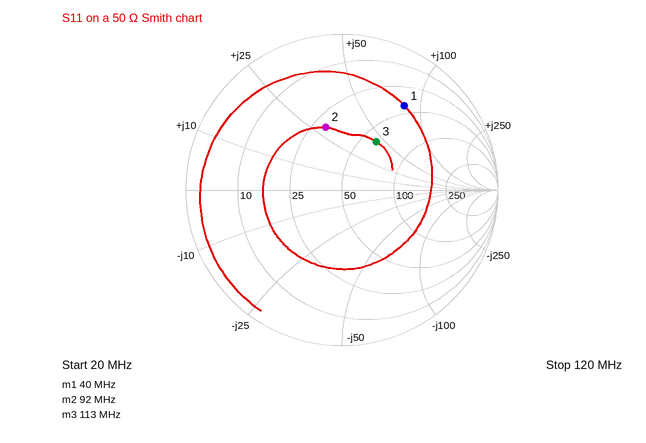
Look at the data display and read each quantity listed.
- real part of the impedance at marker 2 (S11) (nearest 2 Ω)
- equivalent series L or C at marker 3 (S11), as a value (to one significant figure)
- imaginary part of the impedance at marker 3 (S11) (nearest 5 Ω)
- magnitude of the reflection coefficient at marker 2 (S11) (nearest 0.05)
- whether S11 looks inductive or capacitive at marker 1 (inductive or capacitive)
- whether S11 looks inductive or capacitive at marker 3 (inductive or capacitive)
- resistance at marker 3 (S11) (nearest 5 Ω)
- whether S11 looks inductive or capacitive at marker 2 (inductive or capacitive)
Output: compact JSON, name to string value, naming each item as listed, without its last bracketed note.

{"real part of the impedance at marker 2 (S11)": "30 Ω", "equivalent series L or C at marker 3 (S11), as a value": "60 nH", "imaginary part of the impedance at marker 3 (S11)": "+45 Ω", "magnitude of the reflection coefficient at marker 2 (S11)": "0.40", "whether S11 looks inductive or capacitive at marker 1": "inductive", "whether S11 looks inductive or capacitive at marker 3": "inductive", "resistance at marker 3 (S11)": "60 Ω", "whether S11 looks inductive or capacitive at marker 2": "inductive"}
